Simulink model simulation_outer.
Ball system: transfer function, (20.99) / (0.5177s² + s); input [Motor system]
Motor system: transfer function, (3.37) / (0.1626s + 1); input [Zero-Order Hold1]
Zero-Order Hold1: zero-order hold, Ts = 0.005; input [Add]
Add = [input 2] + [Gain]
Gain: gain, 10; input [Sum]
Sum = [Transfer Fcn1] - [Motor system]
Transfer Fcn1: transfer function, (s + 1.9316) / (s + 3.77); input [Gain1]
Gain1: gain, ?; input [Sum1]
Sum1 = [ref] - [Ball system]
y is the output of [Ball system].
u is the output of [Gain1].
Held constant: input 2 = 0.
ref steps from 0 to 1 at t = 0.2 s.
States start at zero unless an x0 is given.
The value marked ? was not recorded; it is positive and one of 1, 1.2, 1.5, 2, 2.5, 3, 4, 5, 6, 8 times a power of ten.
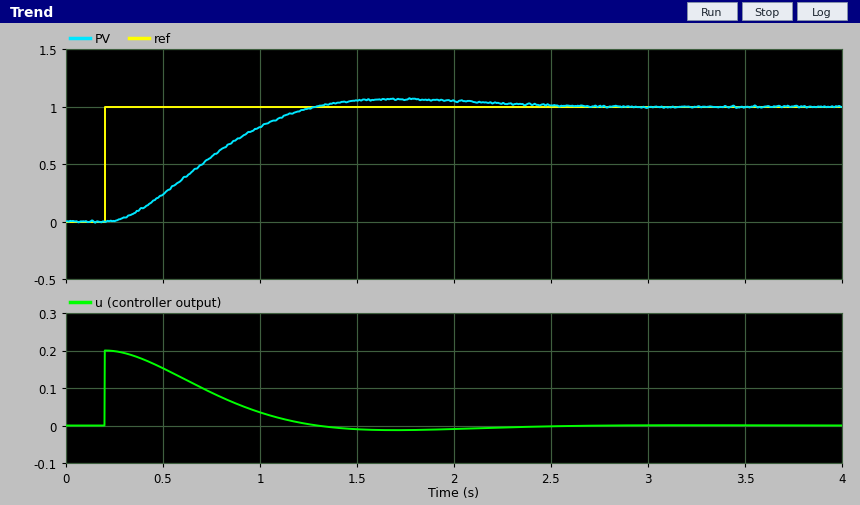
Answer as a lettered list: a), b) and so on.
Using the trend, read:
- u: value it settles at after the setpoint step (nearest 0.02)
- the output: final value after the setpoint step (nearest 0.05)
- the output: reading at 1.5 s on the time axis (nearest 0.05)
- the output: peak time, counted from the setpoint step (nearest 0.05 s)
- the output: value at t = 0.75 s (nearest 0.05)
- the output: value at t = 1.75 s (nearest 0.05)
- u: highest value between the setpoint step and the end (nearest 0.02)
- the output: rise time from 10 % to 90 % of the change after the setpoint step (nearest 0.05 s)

a) 0.00
b) 1.00
c) 1.05
d) 1.50 s
e) 0.55
f) 1.05
g) 0.20
h) 0.70 s
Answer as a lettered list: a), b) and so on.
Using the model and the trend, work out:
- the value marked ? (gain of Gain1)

a) 0.2
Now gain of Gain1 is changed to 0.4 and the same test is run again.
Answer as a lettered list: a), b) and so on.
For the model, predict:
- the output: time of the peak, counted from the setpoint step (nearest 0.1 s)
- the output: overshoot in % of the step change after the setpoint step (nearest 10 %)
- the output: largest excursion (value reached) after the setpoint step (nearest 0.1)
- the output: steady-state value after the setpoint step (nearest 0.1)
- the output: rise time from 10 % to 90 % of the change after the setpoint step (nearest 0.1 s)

a) 0.9 s
b) 20 %
c) 1.2
d) 1.0
e) 0.4 s
